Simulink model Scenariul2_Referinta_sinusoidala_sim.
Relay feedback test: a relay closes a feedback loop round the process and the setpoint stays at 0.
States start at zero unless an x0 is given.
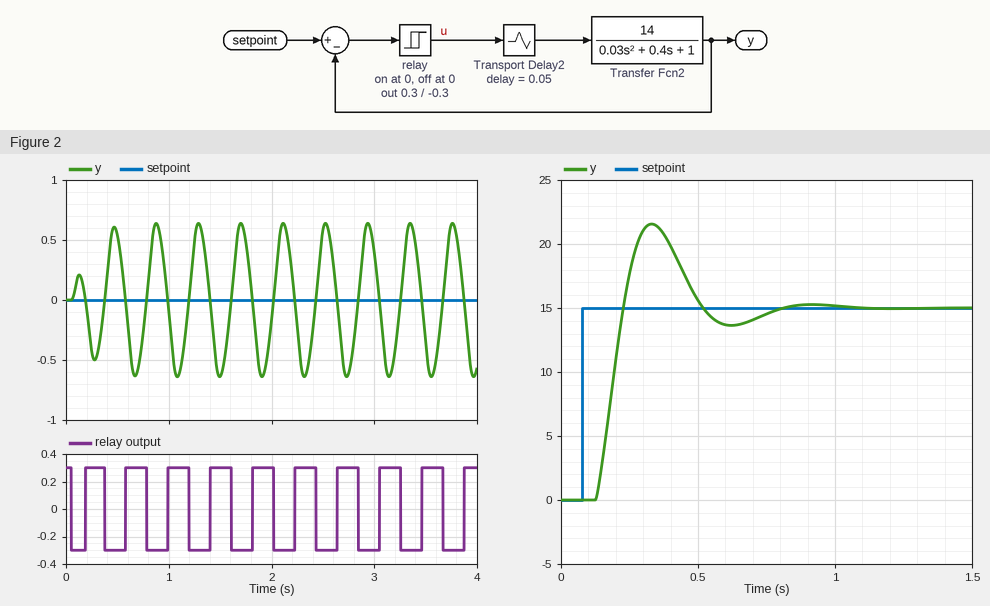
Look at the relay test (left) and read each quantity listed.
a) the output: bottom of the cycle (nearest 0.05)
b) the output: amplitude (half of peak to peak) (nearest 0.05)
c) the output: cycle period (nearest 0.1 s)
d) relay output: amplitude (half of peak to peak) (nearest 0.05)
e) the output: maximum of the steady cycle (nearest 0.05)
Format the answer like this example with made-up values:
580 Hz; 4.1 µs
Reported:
-0.65; 0.65; 0.4 s; 0.30; 0.65
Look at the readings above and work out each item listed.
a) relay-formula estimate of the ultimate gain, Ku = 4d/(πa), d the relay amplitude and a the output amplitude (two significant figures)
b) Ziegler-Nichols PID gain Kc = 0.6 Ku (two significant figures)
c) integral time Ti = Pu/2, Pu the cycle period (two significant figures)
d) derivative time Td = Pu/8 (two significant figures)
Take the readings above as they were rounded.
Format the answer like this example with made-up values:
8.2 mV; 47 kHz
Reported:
0.59; 0.35; 0.20 s; 0.050 s
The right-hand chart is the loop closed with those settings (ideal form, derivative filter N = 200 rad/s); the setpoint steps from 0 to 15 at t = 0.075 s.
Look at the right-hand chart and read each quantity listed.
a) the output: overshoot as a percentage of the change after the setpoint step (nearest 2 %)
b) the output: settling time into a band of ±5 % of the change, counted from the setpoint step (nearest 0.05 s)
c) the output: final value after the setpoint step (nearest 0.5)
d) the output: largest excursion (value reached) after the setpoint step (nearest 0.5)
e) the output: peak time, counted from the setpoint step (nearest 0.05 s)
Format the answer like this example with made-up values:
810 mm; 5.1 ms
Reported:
44 %; 0.65 s; 15.0; 21.5; 0.25 s
